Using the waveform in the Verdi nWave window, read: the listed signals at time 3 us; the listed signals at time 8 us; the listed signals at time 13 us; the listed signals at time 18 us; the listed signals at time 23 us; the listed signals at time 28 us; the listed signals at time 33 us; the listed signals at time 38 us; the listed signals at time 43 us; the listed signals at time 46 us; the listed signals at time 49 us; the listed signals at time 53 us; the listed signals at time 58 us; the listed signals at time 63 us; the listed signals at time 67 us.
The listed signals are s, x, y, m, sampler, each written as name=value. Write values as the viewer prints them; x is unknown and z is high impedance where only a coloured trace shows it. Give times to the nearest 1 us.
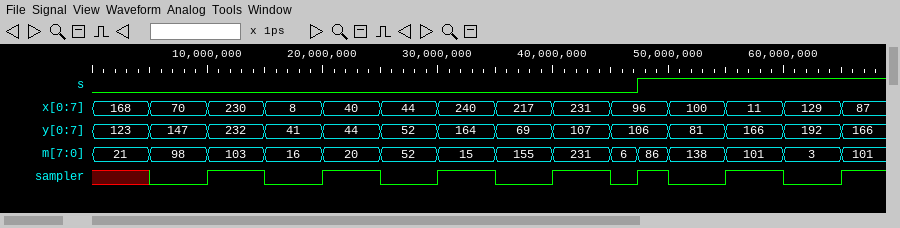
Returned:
s=0, x=168, y=123, m=21, sampler=x
s=0, x=70, y=147, m=98, sampler=0
s=0, x=230, y=232, m=103, sampler=1
s=0, x=8, y=41, m=16, sampler=0
s=0, x=40, y=44, m=20, sampler=1
s=0, x=44, y=52, m=52, sampler=0
s=0, x=240, y=164, m=15, sampler=1
s=0, x=217, y=69, m=155, sampler=0
s=0, x=231, y=107, m=231, sampler=1
s=0, x=96, y=106, m=6, sampler=0
s=1, x=96, y=106, m=86, sampler=1
s=1, x=100, y=81, m=138, sampler=0
s=1, x=11, y=166, m=101, sampler=1
s=1, x=129, y=192, m=3, sampler=0
s=1, x=87, y=166, m=101, sampler=1
